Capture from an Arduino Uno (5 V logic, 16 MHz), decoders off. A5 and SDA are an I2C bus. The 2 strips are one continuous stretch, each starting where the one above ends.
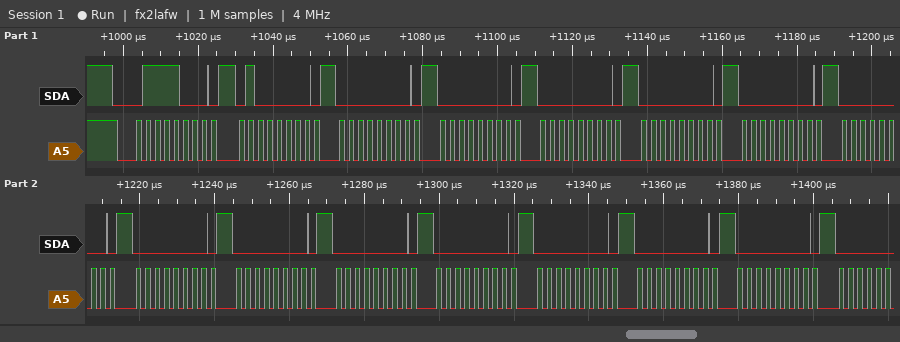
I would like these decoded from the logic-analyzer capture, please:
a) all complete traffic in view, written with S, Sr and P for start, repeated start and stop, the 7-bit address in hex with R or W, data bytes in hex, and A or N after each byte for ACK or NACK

S 3CW A 40 A 00 A 00 A 00 A 00 A 00 A 00 A 00 A 00 A 00 A 00 A 00 A 00 A 00 A
